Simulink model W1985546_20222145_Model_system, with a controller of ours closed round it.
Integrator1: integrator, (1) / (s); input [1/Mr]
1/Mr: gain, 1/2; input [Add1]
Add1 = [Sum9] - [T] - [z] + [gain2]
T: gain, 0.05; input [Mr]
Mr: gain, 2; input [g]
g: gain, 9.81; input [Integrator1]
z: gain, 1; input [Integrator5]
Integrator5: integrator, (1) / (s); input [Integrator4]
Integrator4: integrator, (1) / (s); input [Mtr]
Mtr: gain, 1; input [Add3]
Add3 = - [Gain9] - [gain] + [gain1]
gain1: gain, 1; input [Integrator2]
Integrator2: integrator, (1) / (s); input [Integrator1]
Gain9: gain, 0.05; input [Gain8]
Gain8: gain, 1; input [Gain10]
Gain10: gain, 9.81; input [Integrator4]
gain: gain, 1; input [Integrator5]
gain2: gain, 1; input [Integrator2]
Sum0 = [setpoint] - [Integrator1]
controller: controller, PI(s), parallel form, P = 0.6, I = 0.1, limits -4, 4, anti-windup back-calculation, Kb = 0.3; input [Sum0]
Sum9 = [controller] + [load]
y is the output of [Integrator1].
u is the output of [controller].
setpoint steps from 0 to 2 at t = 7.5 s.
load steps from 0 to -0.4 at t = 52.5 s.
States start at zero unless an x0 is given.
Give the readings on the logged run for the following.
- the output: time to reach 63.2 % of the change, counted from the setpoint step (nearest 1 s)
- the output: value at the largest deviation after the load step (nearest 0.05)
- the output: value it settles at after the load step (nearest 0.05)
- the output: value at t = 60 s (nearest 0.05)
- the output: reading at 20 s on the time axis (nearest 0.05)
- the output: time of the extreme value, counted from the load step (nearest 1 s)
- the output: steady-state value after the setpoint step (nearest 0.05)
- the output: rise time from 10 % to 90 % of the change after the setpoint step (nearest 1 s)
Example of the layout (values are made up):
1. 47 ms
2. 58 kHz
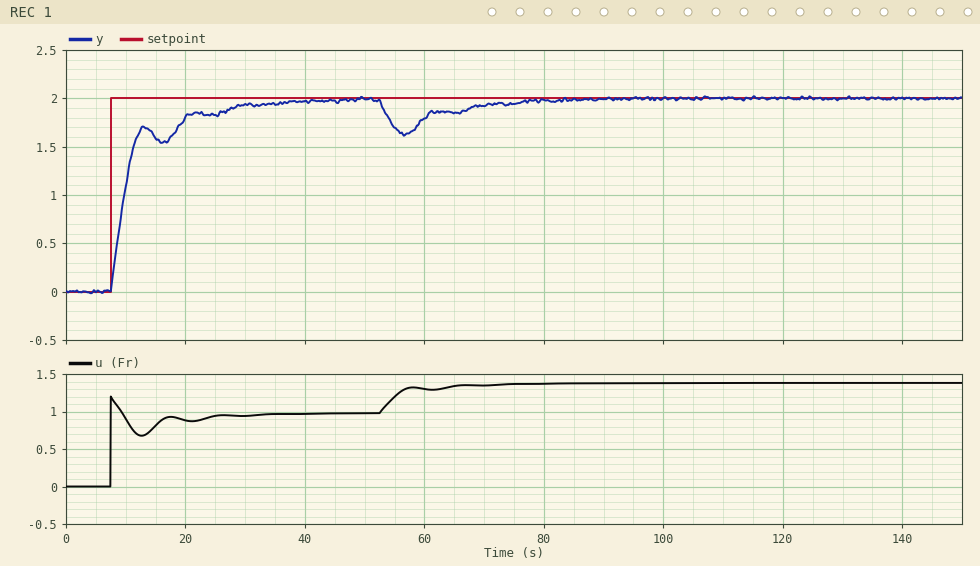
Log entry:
1. 3 s
2. 1.65
3. 2.00
4. 1.80
5. 1.80
6. 4 s
7. 2.00
8. 12 s
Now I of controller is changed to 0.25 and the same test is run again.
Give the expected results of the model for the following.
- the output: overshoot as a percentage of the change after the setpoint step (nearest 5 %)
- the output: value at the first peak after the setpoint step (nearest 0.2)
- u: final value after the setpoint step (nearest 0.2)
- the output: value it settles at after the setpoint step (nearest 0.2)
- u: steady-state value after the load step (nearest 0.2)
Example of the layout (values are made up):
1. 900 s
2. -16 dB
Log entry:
1. 10 %
2. 2.2
3. 1.0
4. 2.0
5. 1.4
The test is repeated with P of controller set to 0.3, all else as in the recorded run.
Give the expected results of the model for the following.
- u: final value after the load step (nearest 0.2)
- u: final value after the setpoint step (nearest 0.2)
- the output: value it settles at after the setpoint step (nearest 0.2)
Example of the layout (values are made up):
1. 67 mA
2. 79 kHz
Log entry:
1. 1.4
2. 1.0
3. 2.0
